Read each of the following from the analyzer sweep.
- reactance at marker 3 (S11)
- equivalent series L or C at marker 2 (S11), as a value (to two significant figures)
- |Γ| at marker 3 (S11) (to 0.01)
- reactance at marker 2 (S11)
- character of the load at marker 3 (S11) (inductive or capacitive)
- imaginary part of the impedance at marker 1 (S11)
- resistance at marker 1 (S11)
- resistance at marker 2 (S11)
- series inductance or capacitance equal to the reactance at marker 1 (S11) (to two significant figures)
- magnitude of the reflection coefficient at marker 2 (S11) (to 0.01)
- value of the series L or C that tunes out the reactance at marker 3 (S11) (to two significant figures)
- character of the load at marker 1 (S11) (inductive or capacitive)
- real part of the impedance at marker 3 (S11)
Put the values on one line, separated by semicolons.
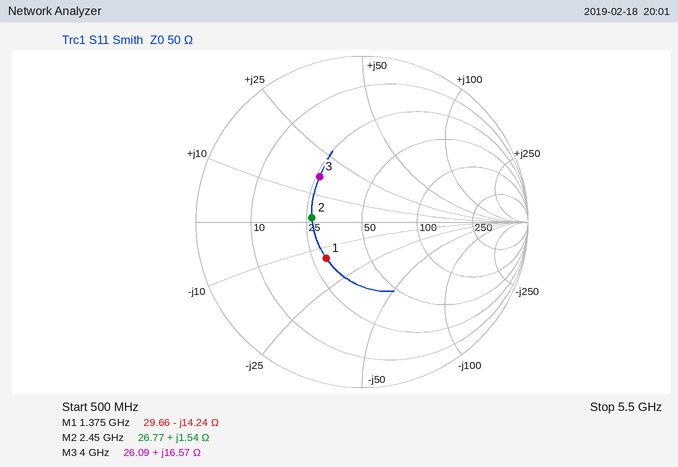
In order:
+16.57 Ω; 100 pH; 0.37; +1.54 Ω; inductive; -14.24 Ω; 29.66 Ω; 26.77 Ω; 8.1 pF; 0.30; 2.4 pF; capacitive; 26.09 Ω
